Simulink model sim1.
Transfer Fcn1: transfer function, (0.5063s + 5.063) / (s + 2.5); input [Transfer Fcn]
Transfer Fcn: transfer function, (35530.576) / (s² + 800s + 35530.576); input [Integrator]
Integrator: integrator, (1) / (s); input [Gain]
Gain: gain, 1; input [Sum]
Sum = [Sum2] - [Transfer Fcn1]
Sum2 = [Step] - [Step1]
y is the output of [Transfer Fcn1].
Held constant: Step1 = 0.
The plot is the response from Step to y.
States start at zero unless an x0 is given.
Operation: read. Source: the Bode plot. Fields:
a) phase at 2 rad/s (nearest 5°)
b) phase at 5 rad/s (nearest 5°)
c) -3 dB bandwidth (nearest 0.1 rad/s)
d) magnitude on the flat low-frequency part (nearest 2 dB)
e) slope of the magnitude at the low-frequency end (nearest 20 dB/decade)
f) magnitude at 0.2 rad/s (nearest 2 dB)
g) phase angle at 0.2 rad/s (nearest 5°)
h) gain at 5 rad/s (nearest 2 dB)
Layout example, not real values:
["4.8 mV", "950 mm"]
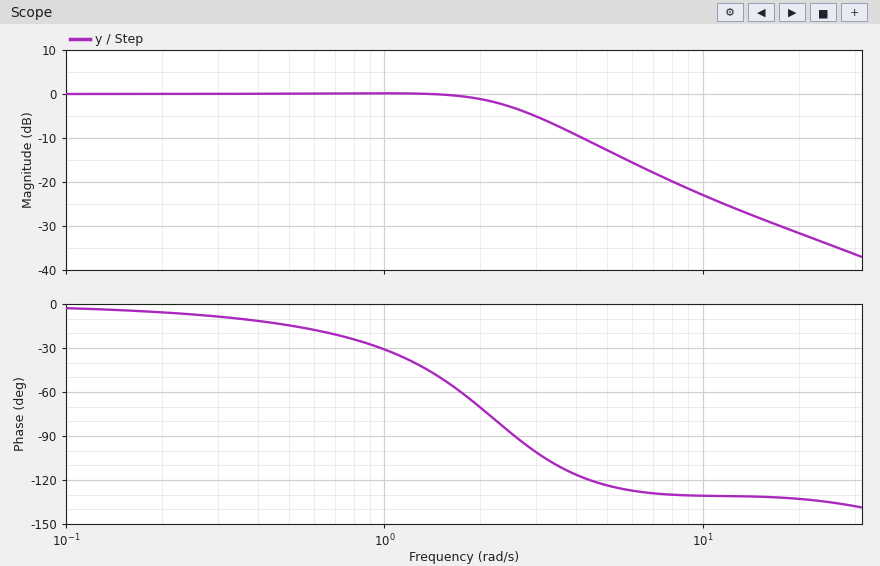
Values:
["-70°", "-125°", "2.5 rad/s", "0 dB", "0 dB/decade", "0 dB", "-5°", "-12 dB"]
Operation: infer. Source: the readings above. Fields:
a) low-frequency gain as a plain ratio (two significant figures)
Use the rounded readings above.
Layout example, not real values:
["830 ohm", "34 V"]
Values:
["1.0"]
